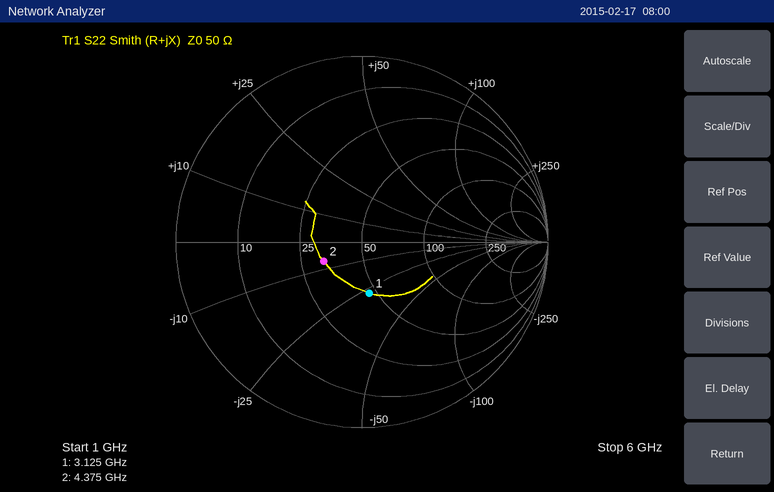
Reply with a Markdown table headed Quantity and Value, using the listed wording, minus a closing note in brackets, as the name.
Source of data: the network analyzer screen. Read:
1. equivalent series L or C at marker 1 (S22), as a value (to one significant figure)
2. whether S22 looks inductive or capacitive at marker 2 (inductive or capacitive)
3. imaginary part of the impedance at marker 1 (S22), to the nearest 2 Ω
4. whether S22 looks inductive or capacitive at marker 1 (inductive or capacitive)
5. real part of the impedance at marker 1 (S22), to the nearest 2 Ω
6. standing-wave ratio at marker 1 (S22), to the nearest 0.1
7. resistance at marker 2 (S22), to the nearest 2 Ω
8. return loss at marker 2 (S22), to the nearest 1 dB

| Quantity | Value |
|---|---|
| equivalent series L or C at marker 1 (S22), as a value | 2 pF |
| whether S22 looks inductive or capacitive at marker 2 | capacitive |
| imaginary part of the impedance at marker 1 (S22), to the nearest 2 Ω | -28 Ω |
| whether S22 looks inductive or capacitive at marker 1 | capacitive |
| real part of the impedance at marker 1 (S22), to the nearest 2 Ω | 46 Ω |
| standing-wave ratio at marker 1 (S22), to the nearest 0.1 | 1.8 |
| resistance at marker 2 (S22), to the nearest 2 Ω | 32 Ω |
| return loss at marker 2 (S22), to the nearest 1 dB | 13 dB |
